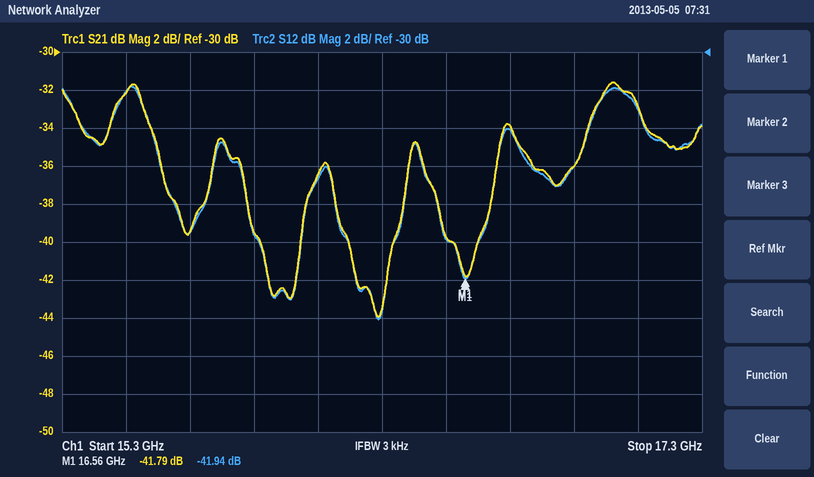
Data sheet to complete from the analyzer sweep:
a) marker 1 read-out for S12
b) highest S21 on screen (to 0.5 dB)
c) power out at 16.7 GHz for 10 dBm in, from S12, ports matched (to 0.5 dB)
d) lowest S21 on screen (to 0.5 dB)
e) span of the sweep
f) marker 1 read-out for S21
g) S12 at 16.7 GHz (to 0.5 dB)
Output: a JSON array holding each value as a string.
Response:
["-41.94 dB", "-31.5 dB", "-24.0 dBm", "-44.0 dB", "2 GHz", "-41.79 dB", "-34.0 dB"]
